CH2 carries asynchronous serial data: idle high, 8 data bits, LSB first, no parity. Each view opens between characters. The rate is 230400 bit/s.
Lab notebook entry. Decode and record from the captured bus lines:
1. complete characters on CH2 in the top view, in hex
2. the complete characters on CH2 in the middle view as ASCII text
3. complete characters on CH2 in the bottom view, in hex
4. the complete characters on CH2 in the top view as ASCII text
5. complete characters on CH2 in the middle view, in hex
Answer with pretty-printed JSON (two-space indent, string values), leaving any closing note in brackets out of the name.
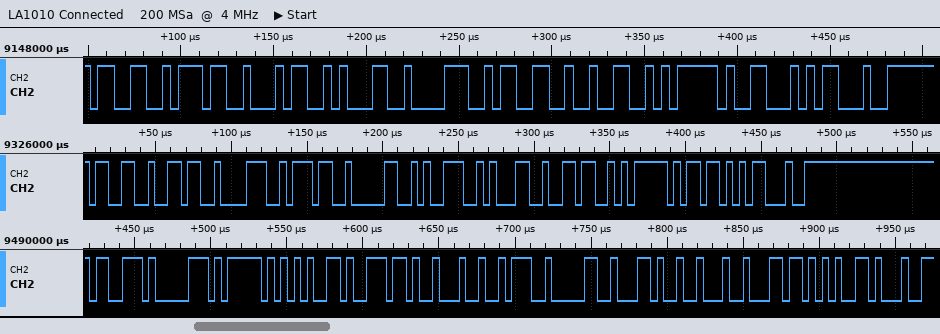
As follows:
{
  "complete characters on CH2 in the top view, in hex": "33, 37, 34, 31, 38, 33, 32, 7D, 46, 23",
  "the complete characters on CH2 in the middle view as ASCII text": "\"36870916}[#\"",
  "complete characters on CH2 in the bottom view, in hex": "73, 70, 5F, 65, 6E, 22, 3A, 30, 2C, 22, 6C, 65",
  "the complete characters on CH2 in the top view as ASCII text": "\"3741832}F#\"",
  "complete characters on CH2 in the middle view, in hex": "33, 36, 38, 37, 30, 39, 31, 36, 7D, 5B, 23"
}
